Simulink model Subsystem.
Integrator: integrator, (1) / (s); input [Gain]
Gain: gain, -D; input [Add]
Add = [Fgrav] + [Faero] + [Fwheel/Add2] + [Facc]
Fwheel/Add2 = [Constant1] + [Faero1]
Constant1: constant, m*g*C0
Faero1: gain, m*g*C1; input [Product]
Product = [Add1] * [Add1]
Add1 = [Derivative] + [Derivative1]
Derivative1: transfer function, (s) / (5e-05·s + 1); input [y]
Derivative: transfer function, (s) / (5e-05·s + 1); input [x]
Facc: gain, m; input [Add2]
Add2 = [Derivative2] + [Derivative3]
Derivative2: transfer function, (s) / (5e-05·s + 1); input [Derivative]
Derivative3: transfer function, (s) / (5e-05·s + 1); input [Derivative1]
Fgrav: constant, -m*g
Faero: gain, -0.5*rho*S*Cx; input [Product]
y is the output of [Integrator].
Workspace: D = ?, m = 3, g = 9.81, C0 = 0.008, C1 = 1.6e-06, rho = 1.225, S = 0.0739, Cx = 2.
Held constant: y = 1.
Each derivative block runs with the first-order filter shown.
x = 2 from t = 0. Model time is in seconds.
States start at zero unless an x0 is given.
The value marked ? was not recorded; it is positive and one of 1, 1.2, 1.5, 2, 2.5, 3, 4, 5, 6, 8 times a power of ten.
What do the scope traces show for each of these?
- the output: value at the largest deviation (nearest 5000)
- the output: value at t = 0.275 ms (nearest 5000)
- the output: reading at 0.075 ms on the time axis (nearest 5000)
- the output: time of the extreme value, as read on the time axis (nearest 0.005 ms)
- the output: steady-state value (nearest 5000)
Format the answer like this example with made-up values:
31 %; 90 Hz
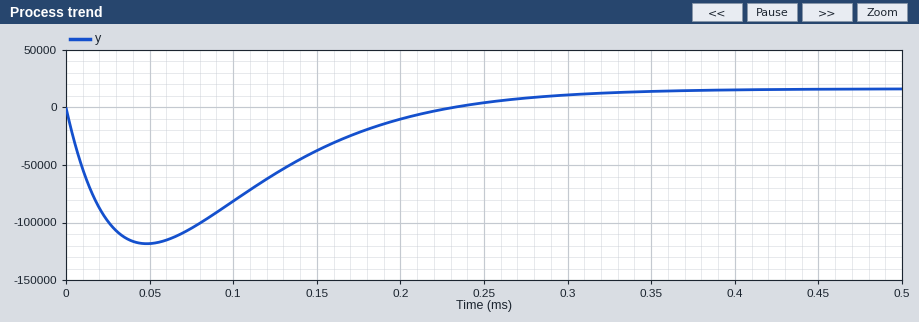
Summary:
-120000; 10000; -105000; 0.050 ms; 15000
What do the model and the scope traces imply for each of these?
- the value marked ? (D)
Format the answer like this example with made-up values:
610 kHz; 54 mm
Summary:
2
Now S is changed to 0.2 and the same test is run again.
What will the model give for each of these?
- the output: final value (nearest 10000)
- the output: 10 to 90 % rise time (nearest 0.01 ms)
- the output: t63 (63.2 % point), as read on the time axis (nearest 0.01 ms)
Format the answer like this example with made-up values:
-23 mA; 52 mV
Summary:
40000; 0.14 ms; 0.23 ms
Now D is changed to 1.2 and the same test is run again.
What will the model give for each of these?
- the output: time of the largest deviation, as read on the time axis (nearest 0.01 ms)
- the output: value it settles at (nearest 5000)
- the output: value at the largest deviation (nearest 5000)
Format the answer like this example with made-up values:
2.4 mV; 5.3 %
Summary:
0.05 ms; 10000; -70000
